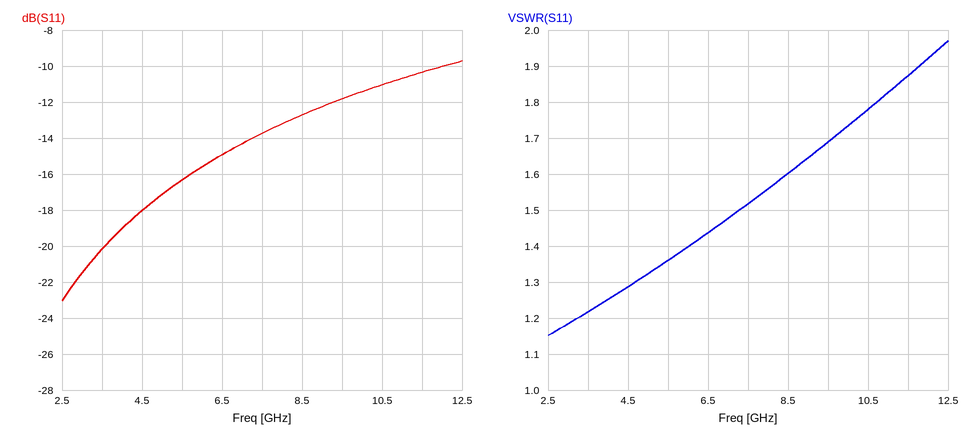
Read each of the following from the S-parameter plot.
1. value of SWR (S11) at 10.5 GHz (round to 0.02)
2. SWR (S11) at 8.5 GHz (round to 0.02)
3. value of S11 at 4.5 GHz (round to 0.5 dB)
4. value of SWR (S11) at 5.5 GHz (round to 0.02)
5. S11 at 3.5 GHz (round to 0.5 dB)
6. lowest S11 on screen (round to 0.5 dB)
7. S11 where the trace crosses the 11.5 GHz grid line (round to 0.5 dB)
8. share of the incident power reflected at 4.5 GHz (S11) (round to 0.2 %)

1.78
1.60
-18.0 dB
1.36
-20.0 dB
-23.0 dB
-10.5 dB
1.6 %
